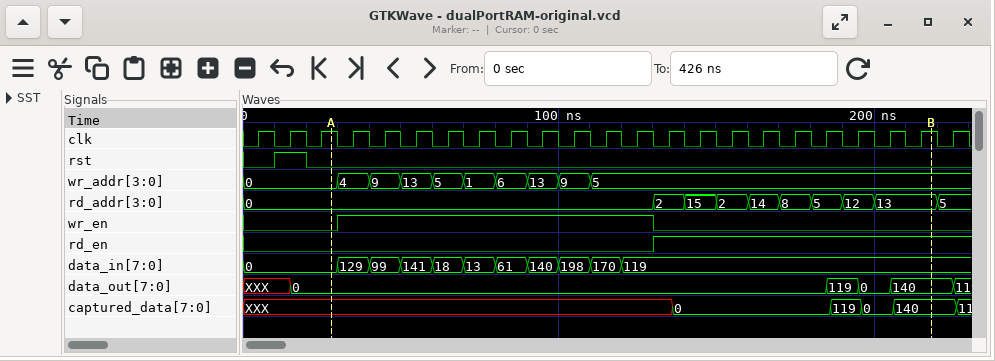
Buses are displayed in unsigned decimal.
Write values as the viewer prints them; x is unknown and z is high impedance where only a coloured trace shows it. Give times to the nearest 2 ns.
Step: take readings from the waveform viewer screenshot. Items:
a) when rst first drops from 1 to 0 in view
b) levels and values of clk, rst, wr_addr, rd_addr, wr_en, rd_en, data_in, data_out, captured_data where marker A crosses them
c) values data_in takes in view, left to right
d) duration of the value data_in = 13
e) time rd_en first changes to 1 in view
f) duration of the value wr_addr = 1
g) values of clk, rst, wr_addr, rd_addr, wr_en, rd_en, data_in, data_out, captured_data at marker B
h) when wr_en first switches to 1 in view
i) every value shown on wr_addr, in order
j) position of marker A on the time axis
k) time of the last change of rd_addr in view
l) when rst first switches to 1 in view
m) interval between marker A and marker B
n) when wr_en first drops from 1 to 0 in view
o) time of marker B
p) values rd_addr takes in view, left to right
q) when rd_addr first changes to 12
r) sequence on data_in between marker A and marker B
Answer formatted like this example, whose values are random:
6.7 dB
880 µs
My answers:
20 ns
clk=1, rst=0, wr_addr=0, rd_addr=0, wr_en=0, rd_en=0, data_in=0, data_out=0, captured_data=XXX
0, 129, 99, 141, 18, 13, 61, 140, 198, 170, 119
10 ns
130 ns
10 ns
clk=1, rst=0, wr_addr=5, rd_addr=13, wr_en=0, rd_en=1, data_in=119, data_out=140, captured_data=140
30 ns
0, 4, 9, 13, 5, 1, 6, 13, 9, 5
28 ns
220 ns
10 ns
190 ns
130 ns
218 ns
0, 2, 15, 2, 14, 8, 5, 12, 13, 5
190 ns
0, 129, 99, 141, 18, 13, 61, 140, 198, 170, 119
